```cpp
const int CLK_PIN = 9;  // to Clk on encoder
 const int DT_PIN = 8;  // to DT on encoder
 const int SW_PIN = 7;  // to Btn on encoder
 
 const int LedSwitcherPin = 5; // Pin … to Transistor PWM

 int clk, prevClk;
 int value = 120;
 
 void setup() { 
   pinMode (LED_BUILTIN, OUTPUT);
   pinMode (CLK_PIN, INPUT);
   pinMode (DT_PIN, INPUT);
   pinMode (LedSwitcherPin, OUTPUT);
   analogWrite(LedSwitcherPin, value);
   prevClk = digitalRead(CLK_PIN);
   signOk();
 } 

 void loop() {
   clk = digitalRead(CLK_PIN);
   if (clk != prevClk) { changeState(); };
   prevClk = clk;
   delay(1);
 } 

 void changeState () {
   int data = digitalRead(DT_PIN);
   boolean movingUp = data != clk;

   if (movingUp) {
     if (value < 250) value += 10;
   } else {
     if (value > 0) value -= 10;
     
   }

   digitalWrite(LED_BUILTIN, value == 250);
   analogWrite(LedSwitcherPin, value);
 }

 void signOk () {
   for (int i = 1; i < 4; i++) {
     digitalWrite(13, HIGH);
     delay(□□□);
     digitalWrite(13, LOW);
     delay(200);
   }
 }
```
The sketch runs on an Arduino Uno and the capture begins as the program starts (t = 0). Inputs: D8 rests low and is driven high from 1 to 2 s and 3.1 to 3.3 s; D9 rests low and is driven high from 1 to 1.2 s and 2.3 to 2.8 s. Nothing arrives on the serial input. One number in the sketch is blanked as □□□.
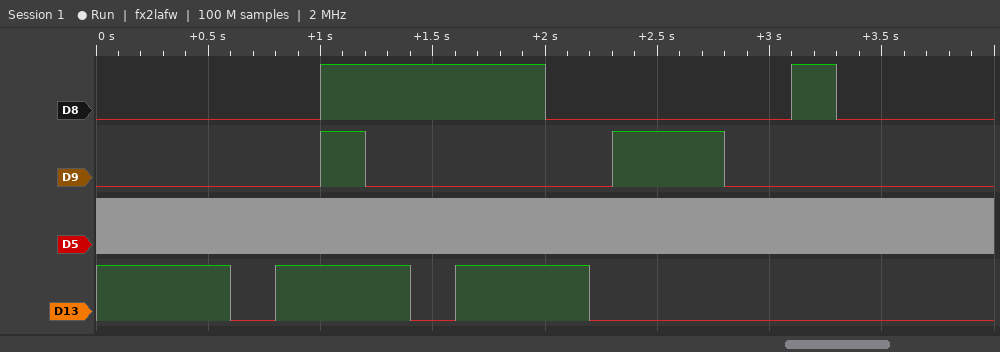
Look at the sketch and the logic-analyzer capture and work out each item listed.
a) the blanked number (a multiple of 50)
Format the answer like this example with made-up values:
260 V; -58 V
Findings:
600
